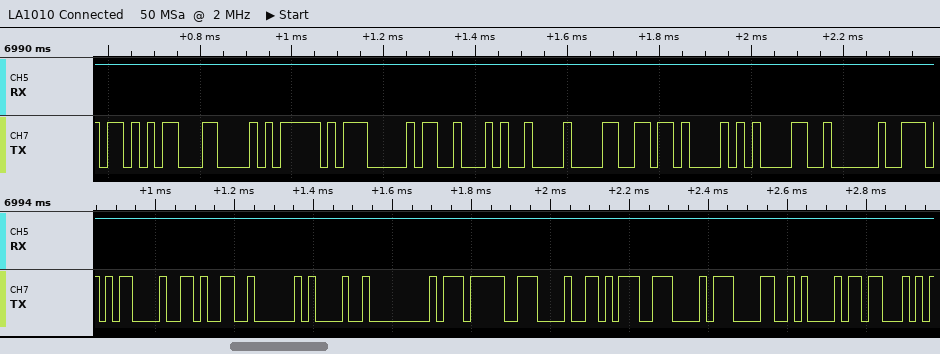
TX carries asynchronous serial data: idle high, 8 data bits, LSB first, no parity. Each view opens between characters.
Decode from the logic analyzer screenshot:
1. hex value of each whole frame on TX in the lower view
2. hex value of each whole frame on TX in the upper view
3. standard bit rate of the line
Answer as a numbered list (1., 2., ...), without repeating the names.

1. 0D, 96, 02, 21, 00, F7, 0E, D6, 0E, 87, 0A, 1B
2. AB, 0C, 7D, 07, 13, 09, 98, 0B, 85, 02
3. 57600 baud
